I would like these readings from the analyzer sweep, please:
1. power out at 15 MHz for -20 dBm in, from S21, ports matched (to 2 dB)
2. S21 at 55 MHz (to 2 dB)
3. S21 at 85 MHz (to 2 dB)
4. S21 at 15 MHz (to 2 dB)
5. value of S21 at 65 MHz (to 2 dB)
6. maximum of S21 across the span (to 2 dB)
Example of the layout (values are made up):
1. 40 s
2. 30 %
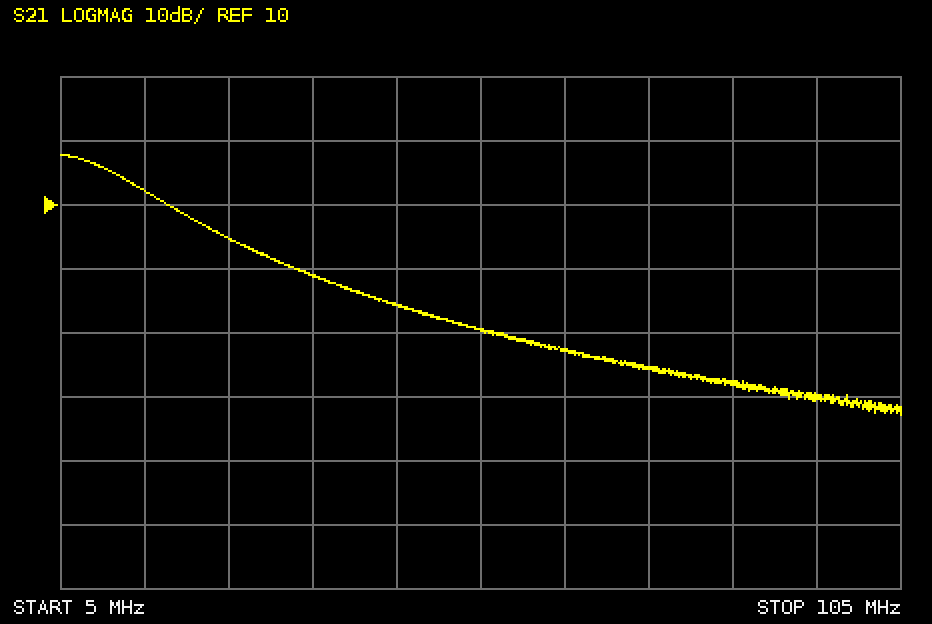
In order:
1. -8 dBm
2. -10 dB
3. -18 dB
4. 12 dB
5. -12 dB
6. 18 dB
